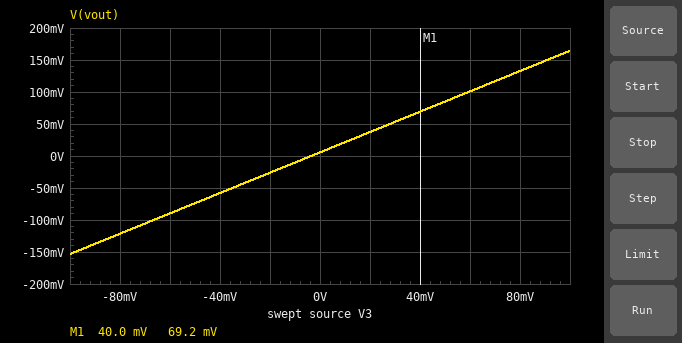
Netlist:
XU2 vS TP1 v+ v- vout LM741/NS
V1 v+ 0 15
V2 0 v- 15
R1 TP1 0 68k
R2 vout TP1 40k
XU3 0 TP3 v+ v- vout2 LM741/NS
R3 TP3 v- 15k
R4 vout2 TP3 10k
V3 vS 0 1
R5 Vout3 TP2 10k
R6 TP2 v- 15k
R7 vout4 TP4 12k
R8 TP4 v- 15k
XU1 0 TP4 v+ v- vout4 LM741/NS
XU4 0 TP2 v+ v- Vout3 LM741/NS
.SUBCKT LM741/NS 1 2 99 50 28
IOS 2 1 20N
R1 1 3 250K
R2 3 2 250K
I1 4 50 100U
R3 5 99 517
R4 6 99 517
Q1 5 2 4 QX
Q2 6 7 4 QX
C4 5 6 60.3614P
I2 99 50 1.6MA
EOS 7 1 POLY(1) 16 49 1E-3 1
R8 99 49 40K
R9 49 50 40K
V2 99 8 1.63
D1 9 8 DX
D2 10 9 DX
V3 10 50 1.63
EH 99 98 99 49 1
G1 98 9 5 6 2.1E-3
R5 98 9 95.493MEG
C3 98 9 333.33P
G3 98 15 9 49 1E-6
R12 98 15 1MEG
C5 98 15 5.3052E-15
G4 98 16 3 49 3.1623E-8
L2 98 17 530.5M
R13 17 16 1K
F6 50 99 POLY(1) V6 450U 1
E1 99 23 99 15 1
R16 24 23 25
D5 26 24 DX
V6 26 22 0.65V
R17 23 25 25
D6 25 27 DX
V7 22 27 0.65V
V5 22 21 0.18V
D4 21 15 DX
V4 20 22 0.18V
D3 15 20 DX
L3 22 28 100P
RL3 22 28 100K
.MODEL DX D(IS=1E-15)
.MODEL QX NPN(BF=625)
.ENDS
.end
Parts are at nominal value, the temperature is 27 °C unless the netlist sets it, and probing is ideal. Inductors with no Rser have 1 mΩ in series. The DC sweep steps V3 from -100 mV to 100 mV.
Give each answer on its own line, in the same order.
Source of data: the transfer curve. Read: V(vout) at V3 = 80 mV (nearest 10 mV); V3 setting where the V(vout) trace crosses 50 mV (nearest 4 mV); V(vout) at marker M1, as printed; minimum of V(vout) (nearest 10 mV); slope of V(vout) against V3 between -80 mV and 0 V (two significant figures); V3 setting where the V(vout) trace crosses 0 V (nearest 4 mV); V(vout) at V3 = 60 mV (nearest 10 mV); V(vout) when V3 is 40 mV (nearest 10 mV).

130 mV
28 mV
69.2 mV
-150 mV
1.6 V/V
-4 mV
100 mV
70 mV
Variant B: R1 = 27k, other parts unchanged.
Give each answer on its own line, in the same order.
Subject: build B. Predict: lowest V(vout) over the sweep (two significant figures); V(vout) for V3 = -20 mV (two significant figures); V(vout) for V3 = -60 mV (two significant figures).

-240 mV
-43 mV
-140 mV
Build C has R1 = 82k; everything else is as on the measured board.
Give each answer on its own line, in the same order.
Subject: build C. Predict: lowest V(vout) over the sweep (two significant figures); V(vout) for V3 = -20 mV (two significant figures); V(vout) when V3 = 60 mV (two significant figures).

-140 mV
-24 mV
95 mV
